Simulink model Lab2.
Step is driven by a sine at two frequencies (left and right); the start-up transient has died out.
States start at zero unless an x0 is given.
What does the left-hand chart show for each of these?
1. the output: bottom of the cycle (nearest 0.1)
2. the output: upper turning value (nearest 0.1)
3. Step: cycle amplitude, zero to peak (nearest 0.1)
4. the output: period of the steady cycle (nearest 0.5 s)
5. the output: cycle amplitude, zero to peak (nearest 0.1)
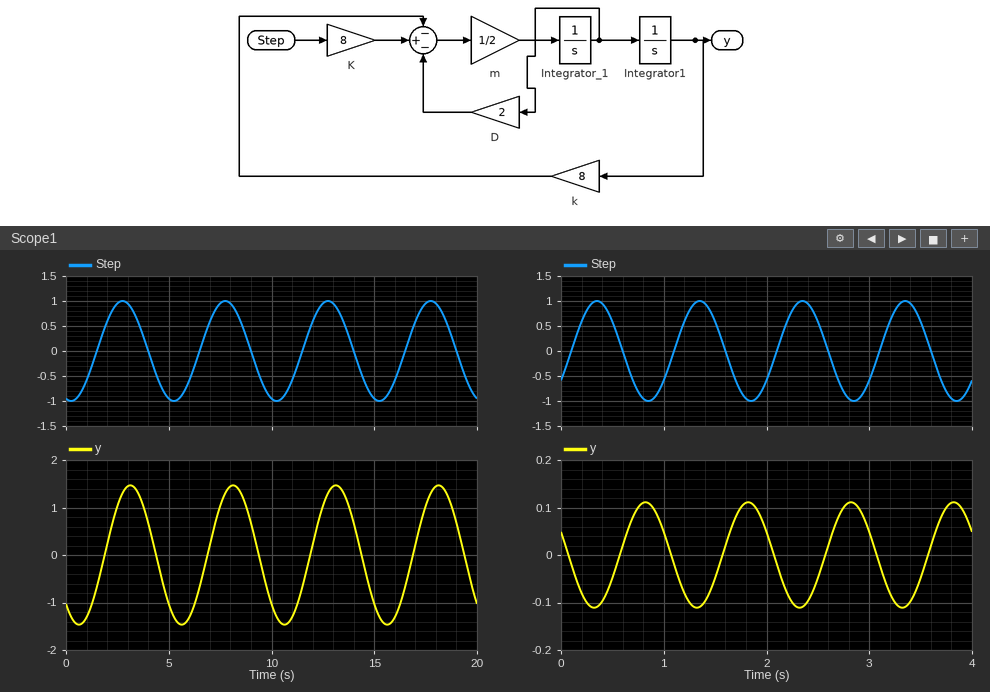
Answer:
-1.5
1.5
1.0
5.0 s
1.5
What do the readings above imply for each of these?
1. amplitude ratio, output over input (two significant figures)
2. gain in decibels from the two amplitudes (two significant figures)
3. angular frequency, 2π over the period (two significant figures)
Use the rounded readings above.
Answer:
1.5
3.5 dB
1.3 rad/s
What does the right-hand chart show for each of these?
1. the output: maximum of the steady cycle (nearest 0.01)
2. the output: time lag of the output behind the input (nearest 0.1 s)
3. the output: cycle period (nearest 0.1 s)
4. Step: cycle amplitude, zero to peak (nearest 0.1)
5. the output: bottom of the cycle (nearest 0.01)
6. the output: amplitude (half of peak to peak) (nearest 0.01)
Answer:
0.11
0.5 s
1.0 s
1.0
-0.11
0.11
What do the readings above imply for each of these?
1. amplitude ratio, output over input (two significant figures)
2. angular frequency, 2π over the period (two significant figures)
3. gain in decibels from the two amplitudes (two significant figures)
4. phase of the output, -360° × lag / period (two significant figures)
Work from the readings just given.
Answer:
0.11
6.3 rad/s
-19 dB
-180°
